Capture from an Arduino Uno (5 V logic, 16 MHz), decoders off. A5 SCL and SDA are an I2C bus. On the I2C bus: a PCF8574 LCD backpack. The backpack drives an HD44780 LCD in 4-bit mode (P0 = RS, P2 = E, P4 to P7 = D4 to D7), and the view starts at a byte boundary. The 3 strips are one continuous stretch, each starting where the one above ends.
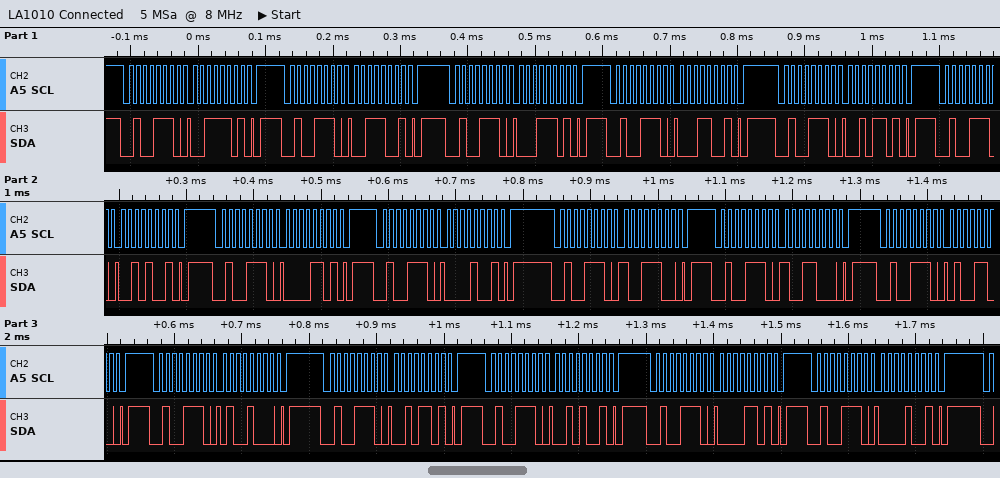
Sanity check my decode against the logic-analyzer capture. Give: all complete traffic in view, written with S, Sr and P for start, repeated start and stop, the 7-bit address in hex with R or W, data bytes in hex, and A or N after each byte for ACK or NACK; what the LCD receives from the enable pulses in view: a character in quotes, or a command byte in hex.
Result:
S 27W A 3D A P S 27W A 39 A P S 27W A 1D A P S 27W A 19 A P S 27W A 2D A P S 27W A 29 A P S 27W A 0D A P S 27W A 09 A P S 27W A 9C A P S 27W A 98 A P S 27W A 4C A P S 27W A 48 A P S 27W A 2D A P S 27W A 29 A P S 27W A 0D A P S 27W A 09 A P
'1' ' ' 0x94 ' '
